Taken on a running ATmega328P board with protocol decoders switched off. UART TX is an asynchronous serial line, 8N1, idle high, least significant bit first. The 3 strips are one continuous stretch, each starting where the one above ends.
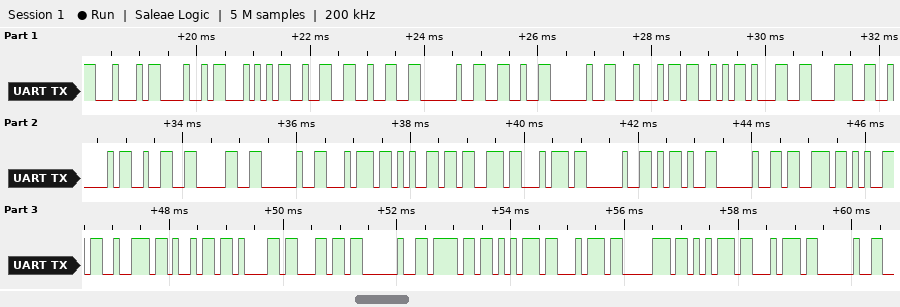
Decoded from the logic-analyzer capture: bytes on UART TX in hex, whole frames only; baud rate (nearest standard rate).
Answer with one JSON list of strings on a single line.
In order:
["0x44 0x48 0x54 0x32 0x32 0x20 0x26 0x20 0x44 0x53 0x31 0x38 0x42 0x32 0x30 0x20 0x74 0x65 0x73 0x74 0x20 0x2D 0x20 0x73 0x65 0x72 0x69 0x61 0x6C 0x20 0x6F 0x75 0x74 0x70 0x75 0x74 0x20", "9600 baud"]
